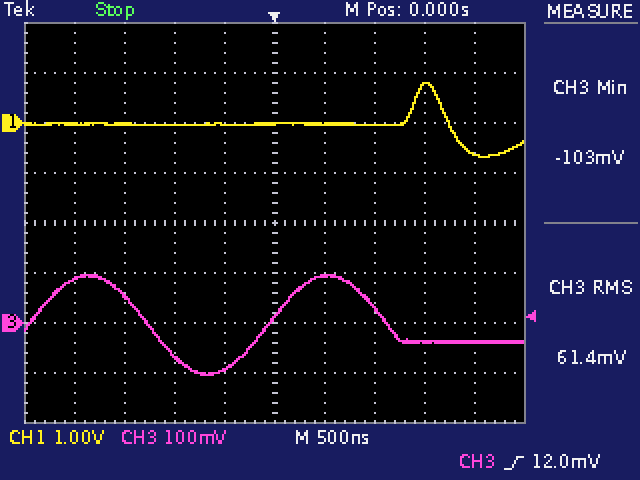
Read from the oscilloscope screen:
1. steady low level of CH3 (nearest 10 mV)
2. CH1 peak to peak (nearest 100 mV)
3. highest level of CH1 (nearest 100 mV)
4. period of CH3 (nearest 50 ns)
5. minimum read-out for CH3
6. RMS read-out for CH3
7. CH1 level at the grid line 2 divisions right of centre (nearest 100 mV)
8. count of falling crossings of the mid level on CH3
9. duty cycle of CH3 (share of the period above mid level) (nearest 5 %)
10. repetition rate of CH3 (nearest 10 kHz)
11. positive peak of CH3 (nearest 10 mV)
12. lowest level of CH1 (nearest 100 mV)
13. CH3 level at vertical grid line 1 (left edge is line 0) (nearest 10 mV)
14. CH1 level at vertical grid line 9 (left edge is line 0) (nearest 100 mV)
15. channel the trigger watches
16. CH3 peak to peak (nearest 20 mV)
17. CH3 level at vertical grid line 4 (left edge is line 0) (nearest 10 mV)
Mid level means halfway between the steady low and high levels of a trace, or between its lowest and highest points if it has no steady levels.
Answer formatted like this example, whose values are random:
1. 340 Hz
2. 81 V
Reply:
1. -40 mV
2. 1.5 V
3. 800 mV
4. 2.40 µs
5. -103 mV
6. 61.4 mV
7. 0.0 V
8. 2
9. 40 %
10. 420 kHz
11. 100 mV
12. -700 mV
13. 90 mV
14. -600 mV
15. CH3
16. 200 mV
17. -90 mV
